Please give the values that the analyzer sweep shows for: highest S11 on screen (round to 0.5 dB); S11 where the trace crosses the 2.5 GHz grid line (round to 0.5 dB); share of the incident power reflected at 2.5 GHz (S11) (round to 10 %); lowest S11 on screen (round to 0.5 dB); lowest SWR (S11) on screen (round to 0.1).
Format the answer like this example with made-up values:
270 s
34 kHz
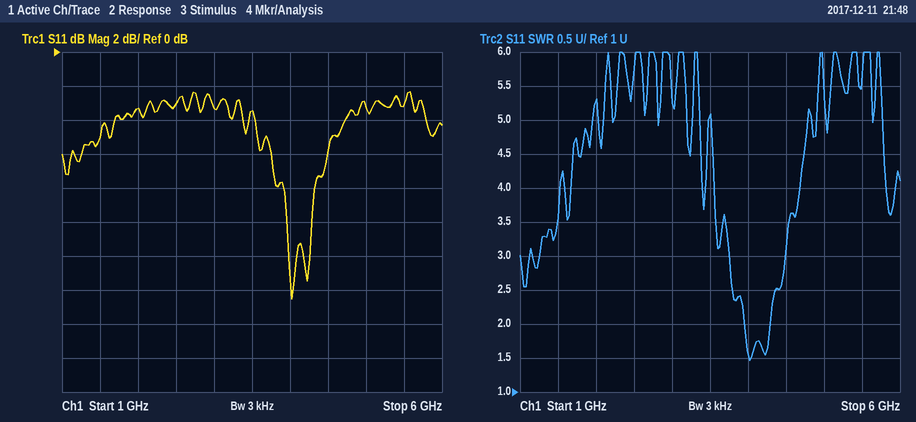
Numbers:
-2.5 dB
-3.0 dB
50 %
-14.5 dB
1.5
